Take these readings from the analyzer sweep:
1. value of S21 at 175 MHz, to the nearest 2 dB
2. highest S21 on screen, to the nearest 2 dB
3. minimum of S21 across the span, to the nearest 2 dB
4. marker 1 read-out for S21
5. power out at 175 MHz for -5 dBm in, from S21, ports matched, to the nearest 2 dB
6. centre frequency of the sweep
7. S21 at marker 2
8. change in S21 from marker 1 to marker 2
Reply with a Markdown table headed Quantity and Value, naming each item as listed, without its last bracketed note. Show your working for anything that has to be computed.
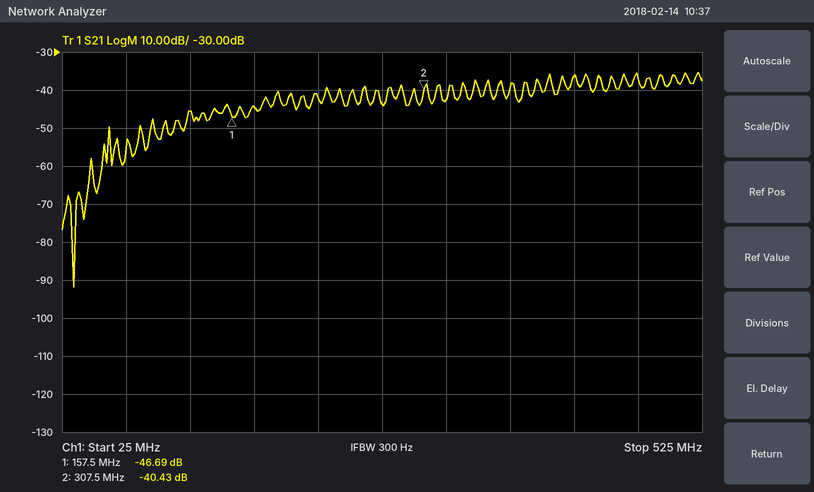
| Quantity | Value |
|---|---|
| value of S21 at 175 MHz, to the nearest 2 dB | -44 dB |
| highest S21 on screen, to the nearest 2 dB | -36 dB |
| minimum of S21 across the span, to the nearest 2 dB | -92 dB |
| marker 1 read-out for S21 | -46.69 dB |
| power out at 175 MHz for -5 dBm in, from S21, ports matched, to the nearest 2 dB | -5 dBm + (-44 dB) = -50 dBm |
| centre frequency of the sweep | 275 MHz |
| S21 at marker 2 | -40.43 dB |
| change in S21 from marker 1 to marker 2 | -40.43 − (-46.69) = 6.26 dB |
